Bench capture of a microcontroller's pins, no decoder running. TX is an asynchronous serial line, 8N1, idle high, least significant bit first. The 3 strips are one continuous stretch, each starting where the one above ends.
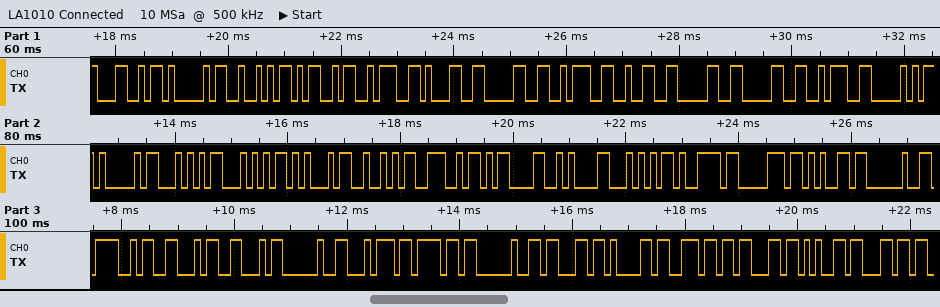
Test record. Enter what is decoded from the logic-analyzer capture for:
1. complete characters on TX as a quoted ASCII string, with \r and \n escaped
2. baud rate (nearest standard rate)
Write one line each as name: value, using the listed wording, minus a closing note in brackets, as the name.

complete characters on TX as a quoted ASCII string, with \r and \n escaped: "LARM:10:200:PATTERN\r\nType OFF to cancel"
baud rate: 9600 baud
